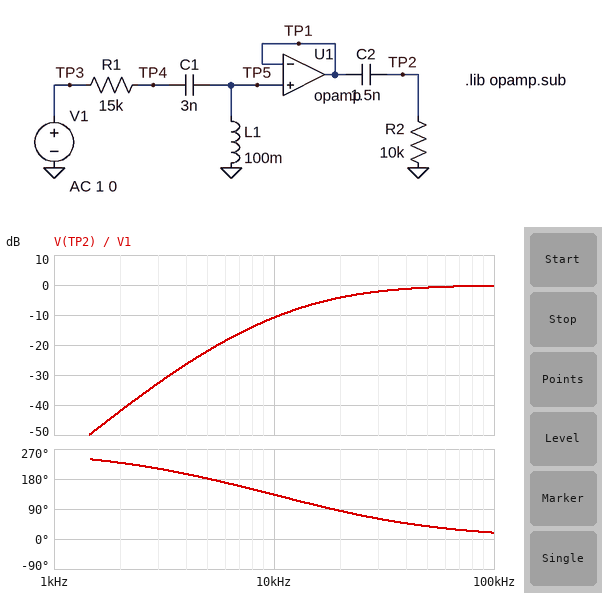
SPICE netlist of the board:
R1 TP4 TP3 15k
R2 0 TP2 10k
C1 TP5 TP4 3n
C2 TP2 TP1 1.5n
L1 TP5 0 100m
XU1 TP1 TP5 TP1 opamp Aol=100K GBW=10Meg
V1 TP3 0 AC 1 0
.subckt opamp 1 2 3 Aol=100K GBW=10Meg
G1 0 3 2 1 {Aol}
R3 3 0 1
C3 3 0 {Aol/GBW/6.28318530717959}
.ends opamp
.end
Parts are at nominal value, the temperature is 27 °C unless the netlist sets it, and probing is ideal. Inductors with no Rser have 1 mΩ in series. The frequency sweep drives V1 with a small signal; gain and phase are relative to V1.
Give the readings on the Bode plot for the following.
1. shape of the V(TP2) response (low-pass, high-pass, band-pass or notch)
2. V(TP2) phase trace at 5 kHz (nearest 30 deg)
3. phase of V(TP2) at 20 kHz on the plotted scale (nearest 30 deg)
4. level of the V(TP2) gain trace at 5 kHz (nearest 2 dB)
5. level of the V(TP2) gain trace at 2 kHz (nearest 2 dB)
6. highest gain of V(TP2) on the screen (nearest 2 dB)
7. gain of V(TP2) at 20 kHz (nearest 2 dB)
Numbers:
high-pass
180 deg
90 deg
-22 dB
-42 dB
0 dB
-4 dB
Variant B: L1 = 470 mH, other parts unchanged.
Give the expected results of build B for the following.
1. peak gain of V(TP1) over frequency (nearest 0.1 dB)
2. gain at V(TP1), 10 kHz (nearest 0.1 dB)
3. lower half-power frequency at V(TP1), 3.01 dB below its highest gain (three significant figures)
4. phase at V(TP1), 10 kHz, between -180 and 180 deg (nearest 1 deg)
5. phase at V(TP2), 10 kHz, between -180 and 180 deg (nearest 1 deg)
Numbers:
0.4 dB
0.3 dB
3.80 kHz
32 deg
78 deg
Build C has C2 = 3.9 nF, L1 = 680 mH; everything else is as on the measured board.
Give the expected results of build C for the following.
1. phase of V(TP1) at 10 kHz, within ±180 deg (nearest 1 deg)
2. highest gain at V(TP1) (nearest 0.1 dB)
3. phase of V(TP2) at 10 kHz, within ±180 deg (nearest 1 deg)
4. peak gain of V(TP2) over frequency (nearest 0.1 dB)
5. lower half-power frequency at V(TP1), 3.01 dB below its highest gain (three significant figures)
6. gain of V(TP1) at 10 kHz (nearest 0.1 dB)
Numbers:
22 deg
1.3 dB
44 deg
0 dB
3.01 kHz
0.5 dB
